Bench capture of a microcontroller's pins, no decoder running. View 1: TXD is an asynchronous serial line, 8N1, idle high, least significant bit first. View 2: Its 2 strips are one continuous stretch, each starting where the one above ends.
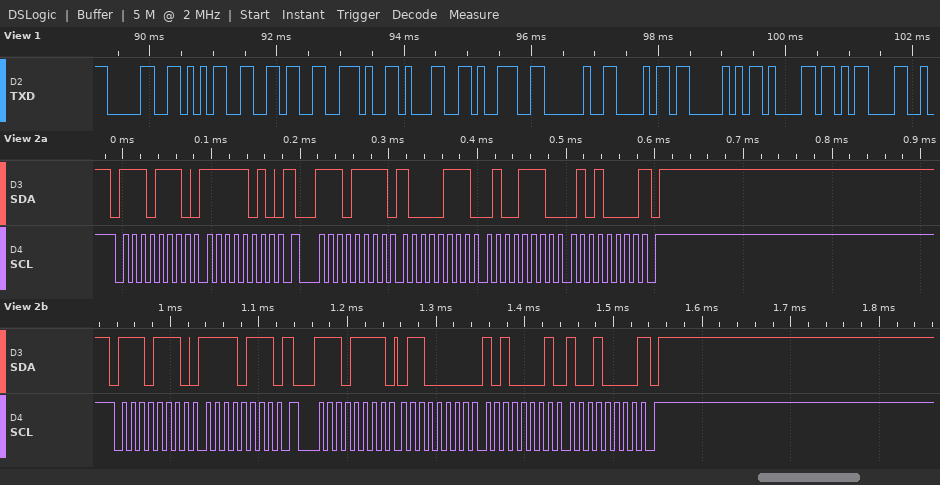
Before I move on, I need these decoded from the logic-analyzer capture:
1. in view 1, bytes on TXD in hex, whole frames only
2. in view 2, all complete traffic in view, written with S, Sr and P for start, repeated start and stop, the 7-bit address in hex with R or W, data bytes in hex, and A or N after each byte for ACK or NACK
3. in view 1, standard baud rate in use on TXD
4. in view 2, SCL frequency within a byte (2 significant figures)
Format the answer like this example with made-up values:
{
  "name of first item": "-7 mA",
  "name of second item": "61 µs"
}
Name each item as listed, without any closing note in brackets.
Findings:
{
  "in view 1, bytes on TXD in hex, whole frames only": "30 35 36 2E 31 39 20 68 50 61 0D",
  "in view 2, all complete traffic in view, written with S, Sr and P for start, repeated start and stop, the 7-bit address in hex with R or W, data bytes in hex, and A or N after each byte for ACK or NACK": "S 77W A FA A Sr 77R A 87 A 4E A 50 N P S 77W A F7 A Sr 77R A 60 A A1 A 90 N P",
  "in view 1, standard baud rate in use on TXD": "9600 baud",
  "in view 2, SCL frequency within a byte": "100 kHz"
}
